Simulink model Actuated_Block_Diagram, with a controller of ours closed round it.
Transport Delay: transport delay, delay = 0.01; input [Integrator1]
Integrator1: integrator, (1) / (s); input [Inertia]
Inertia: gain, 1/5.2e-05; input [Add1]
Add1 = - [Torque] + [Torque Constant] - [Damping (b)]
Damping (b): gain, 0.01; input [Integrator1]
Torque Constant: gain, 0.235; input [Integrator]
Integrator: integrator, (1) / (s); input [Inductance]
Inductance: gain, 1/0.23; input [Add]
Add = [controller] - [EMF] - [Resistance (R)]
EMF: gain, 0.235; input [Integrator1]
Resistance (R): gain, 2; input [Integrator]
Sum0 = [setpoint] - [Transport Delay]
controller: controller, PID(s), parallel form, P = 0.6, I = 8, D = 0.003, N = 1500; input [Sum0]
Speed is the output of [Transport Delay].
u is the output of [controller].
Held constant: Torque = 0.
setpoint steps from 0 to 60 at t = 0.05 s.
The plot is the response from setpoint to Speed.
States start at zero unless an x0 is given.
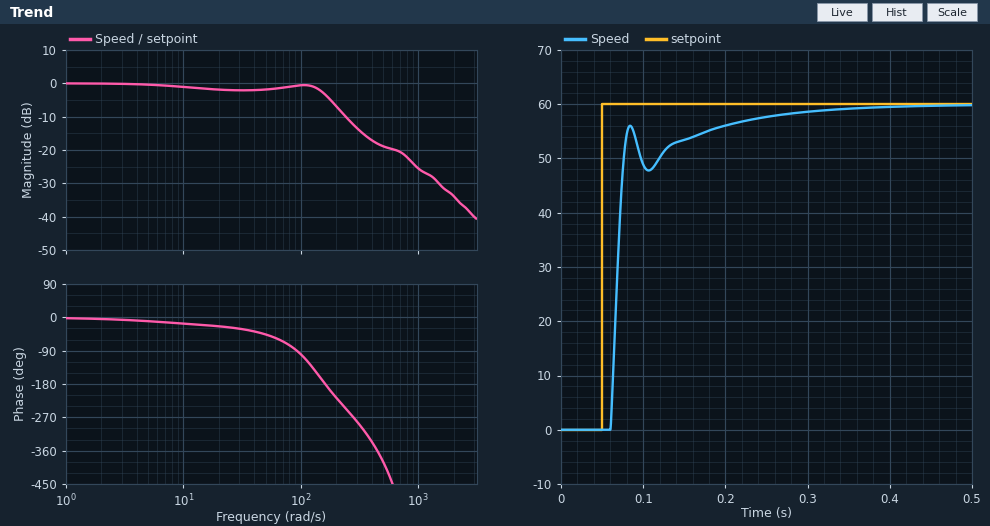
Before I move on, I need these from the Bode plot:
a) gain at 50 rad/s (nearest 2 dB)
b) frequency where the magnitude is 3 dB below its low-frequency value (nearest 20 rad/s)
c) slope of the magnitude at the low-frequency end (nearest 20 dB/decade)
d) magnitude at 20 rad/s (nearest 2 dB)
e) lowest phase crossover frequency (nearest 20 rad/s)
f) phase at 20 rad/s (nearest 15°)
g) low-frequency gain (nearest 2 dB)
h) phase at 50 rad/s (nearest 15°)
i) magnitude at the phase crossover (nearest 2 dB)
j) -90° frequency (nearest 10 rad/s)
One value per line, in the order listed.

-2 dB
160 rad/s
0 dB/decade
-2 dB
160 rad/s
-30°
0 dB
-45°
-4 dB
90 rad/s
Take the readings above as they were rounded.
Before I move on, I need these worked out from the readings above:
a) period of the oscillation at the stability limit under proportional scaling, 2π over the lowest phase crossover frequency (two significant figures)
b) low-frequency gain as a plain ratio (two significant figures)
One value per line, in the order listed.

0.039 s
1.0
